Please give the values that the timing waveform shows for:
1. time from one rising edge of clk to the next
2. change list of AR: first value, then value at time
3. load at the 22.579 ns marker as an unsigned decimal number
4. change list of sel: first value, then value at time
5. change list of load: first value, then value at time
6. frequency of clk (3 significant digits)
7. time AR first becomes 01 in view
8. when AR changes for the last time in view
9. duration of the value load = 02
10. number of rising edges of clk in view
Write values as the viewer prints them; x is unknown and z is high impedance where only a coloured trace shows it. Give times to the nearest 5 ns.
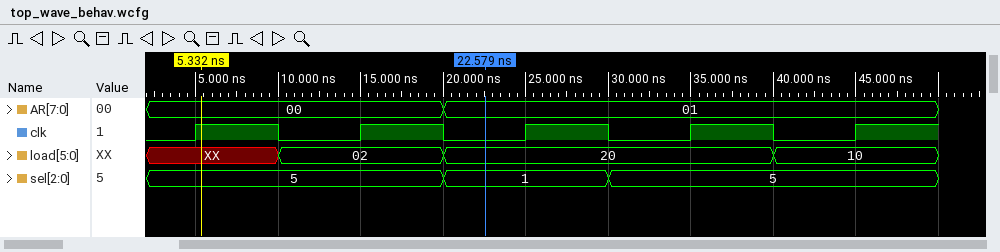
10 ns
00, 01 at 20 ns
32
5, 1 at 20 ns, 5 at 30 ns
XX, 02 at 10 ns, 20 at 20 ns, 10 at 40 ns
100 MHz
20 ns
20 ns
10 ns
5
